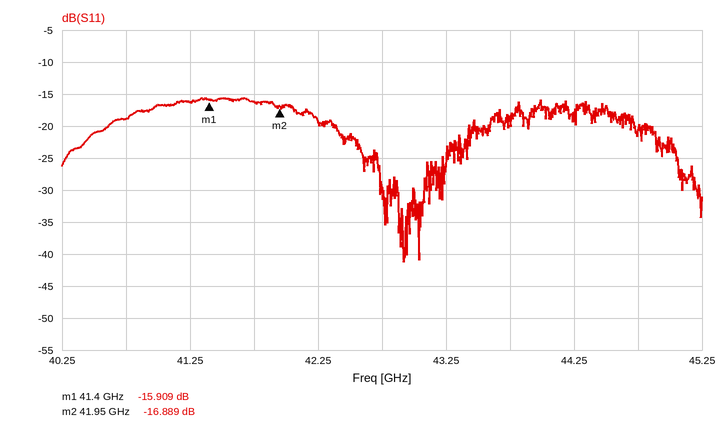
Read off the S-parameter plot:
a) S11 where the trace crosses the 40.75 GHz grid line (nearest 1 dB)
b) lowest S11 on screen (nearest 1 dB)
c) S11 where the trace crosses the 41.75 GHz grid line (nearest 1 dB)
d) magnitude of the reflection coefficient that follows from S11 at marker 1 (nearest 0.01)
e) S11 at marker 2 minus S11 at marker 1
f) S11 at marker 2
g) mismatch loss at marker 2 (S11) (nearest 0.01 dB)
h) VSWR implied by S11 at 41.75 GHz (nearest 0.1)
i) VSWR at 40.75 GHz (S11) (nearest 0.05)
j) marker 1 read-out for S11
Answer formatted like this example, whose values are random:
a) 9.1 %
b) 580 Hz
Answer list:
a) -19 dB
b) -41 dB
c) -16 dB
d) 0.16
e) -0.980 dB
f) -16.889 dB
g) 0.09 dB
h) 1.4
i) 1.25
j) -15.909 dB
